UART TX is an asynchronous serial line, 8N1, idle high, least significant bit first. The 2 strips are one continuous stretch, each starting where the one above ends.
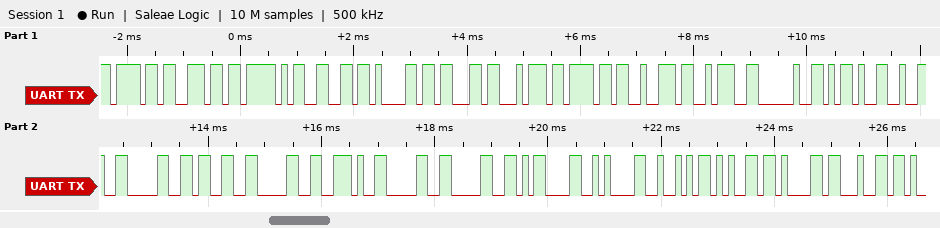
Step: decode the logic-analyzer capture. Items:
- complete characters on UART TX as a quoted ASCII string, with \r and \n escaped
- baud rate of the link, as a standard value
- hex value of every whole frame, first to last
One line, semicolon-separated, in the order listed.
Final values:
"on_factor: -2030.00\r\nRead"; 9600 baud; 6F 6E 5F 66 61 63 74 6F 72 3A 20 2D 32 30 33 30 2E 30 30 0D 0A 52 65 61 64
